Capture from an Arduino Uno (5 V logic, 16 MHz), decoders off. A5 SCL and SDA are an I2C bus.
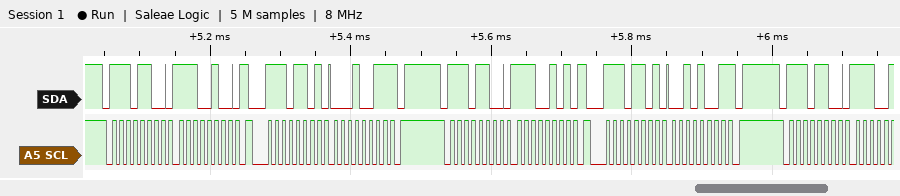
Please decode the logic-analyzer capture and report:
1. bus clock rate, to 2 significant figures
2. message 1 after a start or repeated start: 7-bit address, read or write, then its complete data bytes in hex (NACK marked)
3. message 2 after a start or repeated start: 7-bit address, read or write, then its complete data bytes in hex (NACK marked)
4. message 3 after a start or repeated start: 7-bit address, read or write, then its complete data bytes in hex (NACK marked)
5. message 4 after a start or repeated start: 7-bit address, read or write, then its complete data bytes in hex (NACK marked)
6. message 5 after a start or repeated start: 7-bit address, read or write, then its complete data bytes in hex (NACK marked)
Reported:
100 kHz
0x76 write: E4
0x76 read: 13 NACK
0x76 write: E5
0x76 read: 29 NACK
0x76 write
